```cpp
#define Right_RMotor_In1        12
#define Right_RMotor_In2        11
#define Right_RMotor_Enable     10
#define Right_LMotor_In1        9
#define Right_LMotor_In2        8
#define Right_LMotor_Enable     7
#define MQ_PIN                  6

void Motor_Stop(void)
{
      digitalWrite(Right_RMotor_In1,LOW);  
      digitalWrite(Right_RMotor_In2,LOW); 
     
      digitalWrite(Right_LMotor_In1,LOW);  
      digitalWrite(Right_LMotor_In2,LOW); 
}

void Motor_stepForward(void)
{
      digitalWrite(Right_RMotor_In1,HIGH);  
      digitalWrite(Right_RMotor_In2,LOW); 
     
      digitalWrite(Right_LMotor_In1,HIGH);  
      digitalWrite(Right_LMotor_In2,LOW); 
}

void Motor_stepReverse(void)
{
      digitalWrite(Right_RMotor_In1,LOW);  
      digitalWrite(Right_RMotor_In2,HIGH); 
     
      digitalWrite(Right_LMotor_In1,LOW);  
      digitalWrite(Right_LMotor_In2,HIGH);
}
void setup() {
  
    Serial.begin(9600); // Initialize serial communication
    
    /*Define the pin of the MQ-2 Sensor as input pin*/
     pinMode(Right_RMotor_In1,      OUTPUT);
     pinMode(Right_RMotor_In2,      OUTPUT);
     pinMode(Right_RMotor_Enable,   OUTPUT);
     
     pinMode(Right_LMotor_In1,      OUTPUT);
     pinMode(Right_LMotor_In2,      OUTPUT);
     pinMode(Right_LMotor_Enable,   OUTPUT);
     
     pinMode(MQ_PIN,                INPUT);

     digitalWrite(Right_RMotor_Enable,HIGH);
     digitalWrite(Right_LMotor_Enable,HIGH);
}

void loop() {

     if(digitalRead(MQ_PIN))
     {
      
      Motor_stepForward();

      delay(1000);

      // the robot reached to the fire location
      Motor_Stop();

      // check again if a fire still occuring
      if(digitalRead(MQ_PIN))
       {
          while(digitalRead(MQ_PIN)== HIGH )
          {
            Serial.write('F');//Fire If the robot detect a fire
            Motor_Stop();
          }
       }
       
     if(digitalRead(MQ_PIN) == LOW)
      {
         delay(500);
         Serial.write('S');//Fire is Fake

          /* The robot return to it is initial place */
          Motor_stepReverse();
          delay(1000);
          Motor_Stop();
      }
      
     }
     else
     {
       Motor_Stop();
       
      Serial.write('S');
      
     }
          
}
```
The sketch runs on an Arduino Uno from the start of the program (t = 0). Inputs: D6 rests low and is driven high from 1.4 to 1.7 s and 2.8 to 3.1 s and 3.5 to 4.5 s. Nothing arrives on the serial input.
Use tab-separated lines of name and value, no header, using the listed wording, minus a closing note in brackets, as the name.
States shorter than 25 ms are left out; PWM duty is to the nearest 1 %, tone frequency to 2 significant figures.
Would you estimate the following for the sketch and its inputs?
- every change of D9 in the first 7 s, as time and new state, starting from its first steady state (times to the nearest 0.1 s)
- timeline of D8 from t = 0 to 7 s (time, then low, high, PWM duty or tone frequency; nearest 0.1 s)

every change of D9 in the first 7 s, as time and new state, starting from its first steady state	0 s low; 1.4 s high; 2.4 s low; 3.9 s high; 4.9 s low
timeline of D8 from t = 0 to 7 s	0 s low; 2.9 s high; 3.9 s low; 5.4 s high; 6.4 s low
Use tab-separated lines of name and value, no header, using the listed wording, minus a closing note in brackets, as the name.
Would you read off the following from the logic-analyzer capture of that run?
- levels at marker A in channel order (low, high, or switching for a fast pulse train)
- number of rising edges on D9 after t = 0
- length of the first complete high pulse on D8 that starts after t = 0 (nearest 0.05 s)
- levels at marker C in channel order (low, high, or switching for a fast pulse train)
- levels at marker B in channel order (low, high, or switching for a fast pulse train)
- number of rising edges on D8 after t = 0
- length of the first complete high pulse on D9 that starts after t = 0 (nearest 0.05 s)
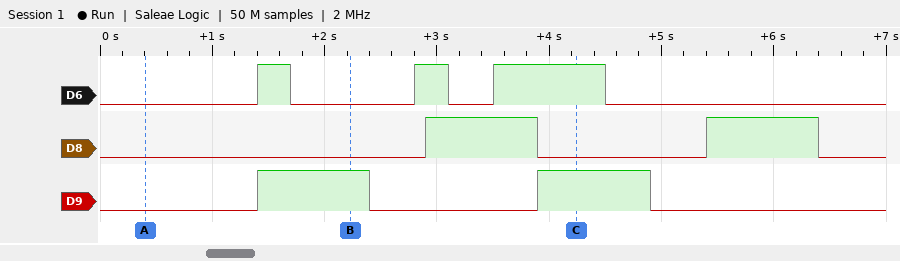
levels at marker A in channel order	D6 low, D8 low, D9 low
number of rising edges on D9 after t = 0	2
length of the first complete high pulse on D8 that starts after t = 0	1.00 s
levels at marker C in channel order	D6 high, D8 low, D9 high
levels at marker B in channel order	D6 low, D8 low, D9 high
number of rising edges on D8 after t = 0	2
length of the first complete high pulse on D9 that starts after t = 0	1.00 s
